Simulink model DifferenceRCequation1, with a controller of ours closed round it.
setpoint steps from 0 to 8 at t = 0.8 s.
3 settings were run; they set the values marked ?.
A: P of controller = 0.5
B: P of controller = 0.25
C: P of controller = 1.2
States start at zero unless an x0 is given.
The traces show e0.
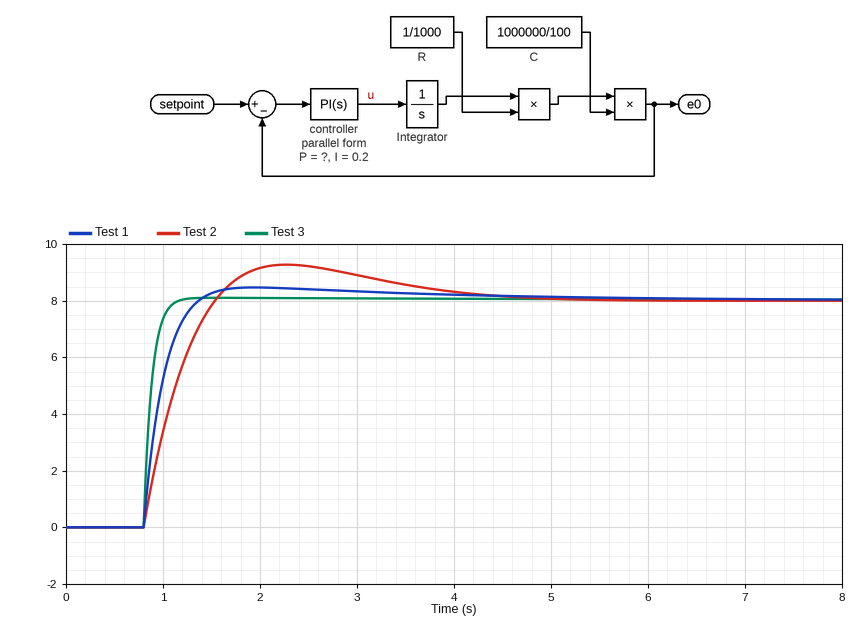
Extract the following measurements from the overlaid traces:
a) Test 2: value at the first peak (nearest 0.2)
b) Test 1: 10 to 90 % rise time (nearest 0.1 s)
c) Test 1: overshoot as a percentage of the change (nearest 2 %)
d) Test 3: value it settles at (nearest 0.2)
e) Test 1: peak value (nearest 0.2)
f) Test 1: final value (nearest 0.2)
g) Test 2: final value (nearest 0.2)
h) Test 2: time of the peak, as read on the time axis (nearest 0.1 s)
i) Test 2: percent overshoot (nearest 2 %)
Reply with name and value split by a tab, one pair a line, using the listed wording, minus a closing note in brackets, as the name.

Test 2: value at the first peak	9.2
Test 1: 10 to 90 % rise time	0.4 s
Test 1: overshoot as a percentage of the change	6 %
Test 3: value it settles at	8.0
Test 1: peak value	8.4
Test 1: final value	8.0
Test 2: final value	8.0
Test 2: time of the peak, as read on the time axis	2.3 s
Test 2: percent overshoot	16 %
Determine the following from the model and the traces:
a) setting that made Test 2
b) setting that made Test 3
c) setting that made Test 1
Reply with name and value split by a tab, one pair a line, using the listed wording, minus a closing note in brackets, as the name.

setting that made Test 2	B
setting that made Test 3	C
setting that made Test 1	A
